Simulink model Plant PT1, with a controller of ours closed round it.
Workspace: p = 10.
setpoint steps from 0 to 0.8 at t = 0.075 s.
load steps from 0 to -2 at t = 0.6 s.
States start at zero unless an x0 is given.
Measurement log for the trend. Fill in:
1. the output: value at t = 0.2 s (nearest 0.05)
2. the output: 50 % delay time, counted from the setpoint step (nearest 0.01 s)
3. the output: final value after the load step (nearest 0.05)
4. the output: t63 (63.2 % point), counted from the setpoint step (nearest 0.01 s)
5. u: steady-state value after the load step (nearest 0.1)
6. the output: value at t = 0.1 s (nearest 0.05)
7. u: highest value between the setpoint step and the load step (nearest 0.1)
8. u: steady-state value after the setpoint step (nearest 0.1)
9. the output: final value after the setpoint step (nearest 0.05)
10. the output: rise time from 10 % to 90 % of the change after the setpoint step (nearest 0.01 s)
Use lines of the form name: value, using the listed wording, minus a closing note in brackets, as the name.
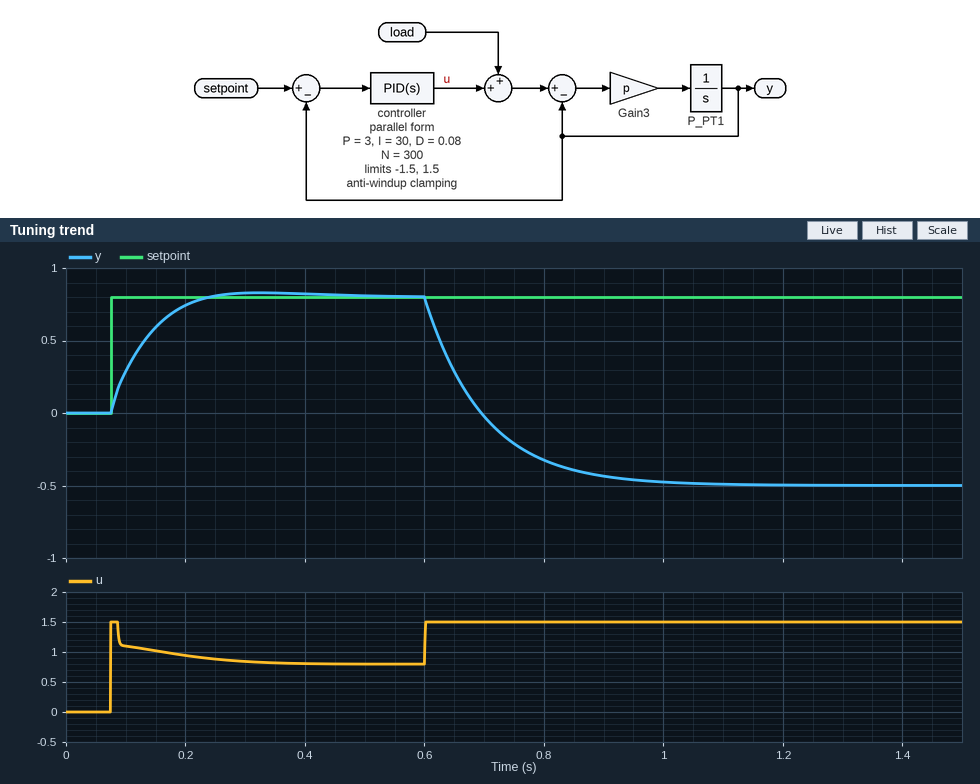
the output: value at t = 0.2 s: 0.75
the output: 50 % delay time, counted from the setpoint step: 0.04 s
the output: final value after the load step: -0.50
the output: t63 (63.2 % point), counted from the setpoint step: 0.06 s
u: steady-state value after the load step: 1.5
the output: value at t = 0.1 s: 0.30
u: highest value between the setpoint step and the load step: 1.5
u: steady-state value after the setpoint step: 0.8
the output: final value after the setpoint step: 0.80
the output: rise time from 10 % to 90 % of the change after the setpoint step: 0.11 s
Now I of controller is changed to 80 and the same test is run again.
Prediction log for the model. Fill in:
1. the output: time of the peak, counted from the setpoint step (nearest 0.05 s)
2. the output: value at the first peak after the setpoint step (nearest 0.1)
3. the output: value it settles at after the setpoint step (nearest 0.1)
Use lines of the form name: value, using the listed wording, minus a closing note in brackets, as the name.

the output: time of the peak, counted from the setpoint step: 0.15 s
the output: value at the first peak after the setpoint step: 0.9
the output: value it settles at after the setpoint step: 0.8
